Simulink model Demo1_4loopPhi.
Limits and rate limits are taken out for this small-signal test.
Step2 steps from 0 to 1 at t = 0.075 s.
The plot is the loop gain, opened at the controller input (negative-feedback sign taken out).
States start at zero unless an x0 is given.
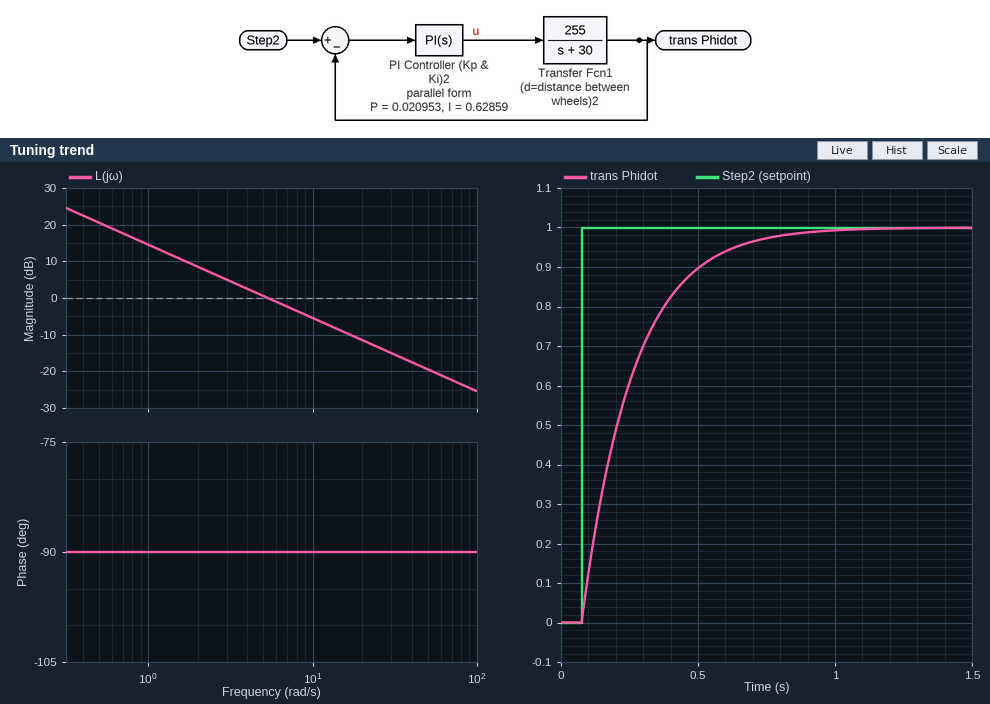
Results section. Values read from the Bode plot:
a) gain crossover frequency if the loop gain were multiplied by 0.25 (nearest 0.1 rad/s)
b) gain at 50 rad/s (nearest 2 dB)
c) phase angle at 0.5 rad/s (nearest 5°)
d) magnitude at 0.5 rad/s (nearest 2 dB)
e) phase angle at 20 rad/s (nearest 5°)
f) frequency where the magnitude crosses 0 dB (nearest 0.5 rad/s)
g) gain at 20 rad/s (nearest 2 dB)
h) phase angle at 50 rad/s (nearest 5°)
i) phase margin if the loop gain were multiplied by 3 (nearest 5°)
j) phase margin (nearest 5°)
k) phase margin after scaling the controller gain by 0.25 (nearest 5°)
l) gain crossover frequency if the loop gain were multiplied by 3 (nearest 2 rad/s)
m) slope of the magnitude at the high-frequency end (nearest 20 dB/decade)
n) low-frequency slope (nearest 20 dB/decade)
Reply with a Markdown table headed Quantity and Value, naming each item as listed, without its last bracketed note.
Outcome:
| Quantity | Value |
|---|---|
| gain crossover frequency if the loop gain were multiplied by 0.25 | 1.3 rad/s |
| gain at 50 rad/s | -20 dB |
| phase angle at 0.5 rad/s | -90° |
| magnitude at 0.5 rad/s | 20 dB |
| phase angle at 20 rad/s | -90° |
| frequency where the magnitude crosses 0 dB | 5.5 rad/s |
| gain at 20 rad/s | -12 dB |
| phase angle at 50 rad/s | -90° |
| phase margin if the loop gain were multiplied by 3 | 90° |
| phase margin | 90° |
| phase margin after scaling the controller gain by 0.25 | 90° |
| gain crossover frequency if the loop gain were multiplied by 3 | 16 rad/s |
| slope of the magnitude at the high-frequency end | -20 dB/decade |
| low-frequency slope | -20 dB/decade |
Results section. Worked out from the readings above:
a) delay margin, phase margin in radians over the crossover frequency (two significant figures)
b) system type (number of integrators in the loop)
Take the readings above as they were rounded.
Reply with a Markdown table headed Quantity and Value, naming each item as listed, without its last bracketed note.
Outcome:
| Quantity | Value |
|---|---|
| delay margin, phase margin in radians over the crossover frequency | 0.29 s |
| system type | 1 |
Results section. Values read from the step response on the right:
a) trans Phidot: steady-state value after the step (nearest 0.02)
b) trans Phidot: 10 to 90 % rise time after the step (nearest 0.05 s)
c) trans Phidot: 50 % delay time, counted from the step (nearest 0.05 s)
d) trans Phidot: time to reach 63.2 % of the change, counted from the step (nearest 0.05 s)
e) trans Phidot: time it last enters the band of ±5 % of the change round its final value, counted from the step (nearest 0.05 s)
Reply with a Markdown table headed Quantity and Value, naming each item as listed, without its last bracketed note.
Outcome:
| Quantity | Value |
|---|---|
| trans Phidot: steady-state value after the step | 1.00 |
| trans Phidot: 10 to 90 % rise time after the step | 0.40 s |
| trans Phidot: 50 % delay time, counted from the step | 0.15 s |
| trans Phidot: time to reach 63.2 % of the change, counted from the step | 0.20 s |
| trans Phidot: time it last enters the band of ±5 % of the change round its final value, counted from the step | 0.55 s |
